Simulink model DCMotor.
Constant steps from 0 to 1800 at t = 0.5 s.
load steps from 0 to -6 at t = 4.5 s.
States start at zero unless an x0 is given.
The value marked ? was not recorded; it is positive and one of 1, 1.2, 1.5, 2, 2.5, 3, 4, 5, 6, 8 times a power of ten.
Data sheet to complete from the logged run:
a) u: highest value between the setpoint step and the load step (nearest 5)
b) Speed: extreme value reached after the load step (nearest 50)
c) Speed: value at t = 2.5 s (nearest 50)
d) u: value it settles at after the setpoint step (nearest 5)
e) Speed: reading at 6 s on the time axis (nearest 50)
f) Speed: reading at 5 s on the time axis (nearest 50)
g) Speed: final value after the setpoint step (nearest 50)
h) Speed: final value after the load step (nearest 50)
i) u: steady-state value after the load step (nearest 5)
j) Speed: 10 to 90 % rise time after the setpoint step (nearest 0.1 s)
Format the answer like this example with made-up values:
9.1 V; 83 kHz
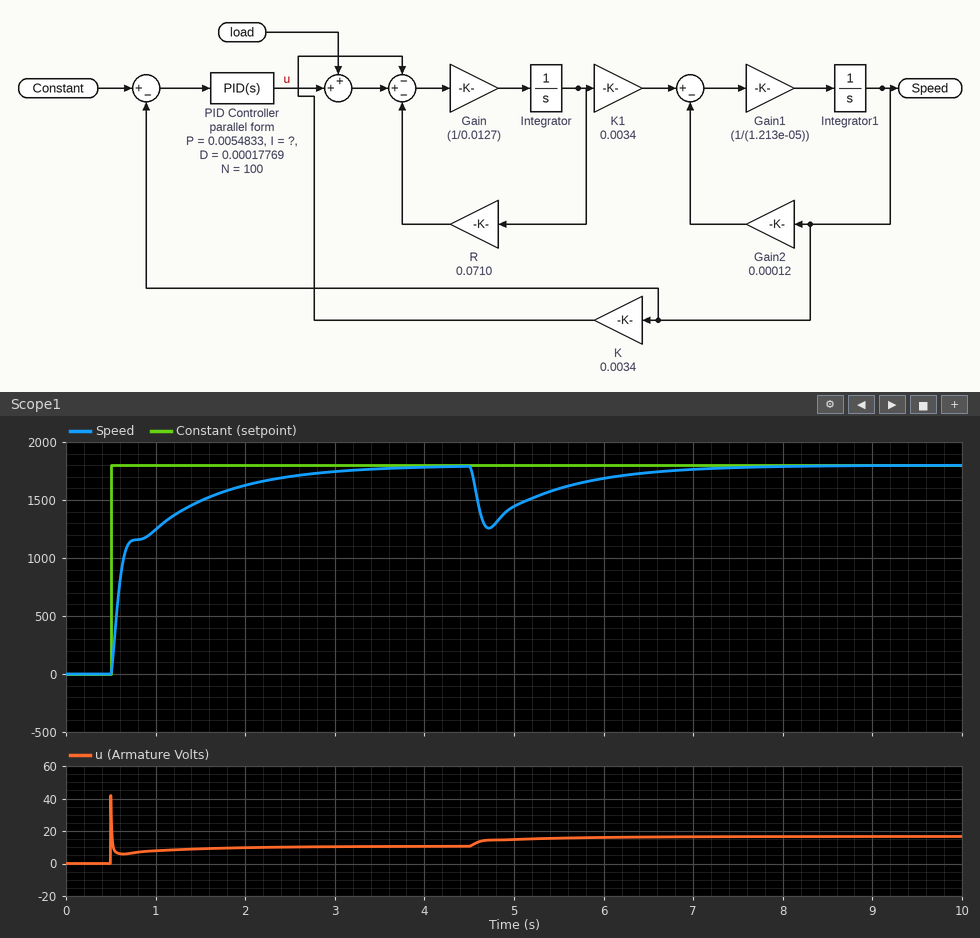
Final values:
40; 1250; 1700; 10; 1700; 1450; 1800; 1800; 15; 1.4 s
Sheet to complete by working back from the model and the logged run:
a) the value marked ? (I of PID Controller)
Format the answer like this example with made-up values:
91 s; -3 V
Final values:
0.012
